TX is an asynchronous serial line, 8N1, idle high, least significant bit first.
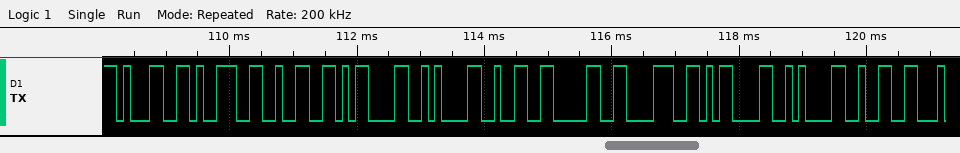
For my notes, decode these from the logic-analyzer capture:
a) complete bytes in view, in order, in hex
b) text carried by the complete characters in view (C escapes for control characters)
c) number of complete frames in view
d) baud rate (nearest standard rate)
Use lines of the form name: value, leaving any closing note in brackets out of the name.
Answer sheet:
complete bytes in view, in order, in hex: 0x31 0x39 0x32 0x0D 0x0A 0x32 0x30 0x38 0x0D 0x0A 0x32
text carried by the complete characters in view: "192\r\n208\r\n2"
number of complete frames in view: 11
baud rate: 9600 baud
